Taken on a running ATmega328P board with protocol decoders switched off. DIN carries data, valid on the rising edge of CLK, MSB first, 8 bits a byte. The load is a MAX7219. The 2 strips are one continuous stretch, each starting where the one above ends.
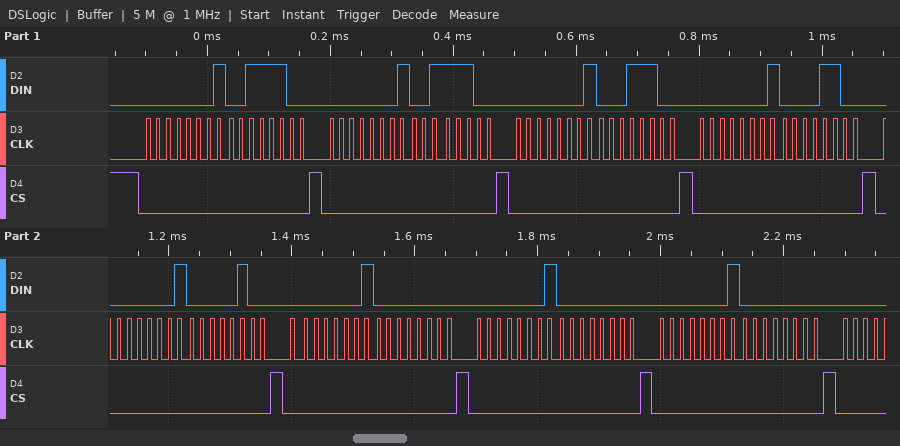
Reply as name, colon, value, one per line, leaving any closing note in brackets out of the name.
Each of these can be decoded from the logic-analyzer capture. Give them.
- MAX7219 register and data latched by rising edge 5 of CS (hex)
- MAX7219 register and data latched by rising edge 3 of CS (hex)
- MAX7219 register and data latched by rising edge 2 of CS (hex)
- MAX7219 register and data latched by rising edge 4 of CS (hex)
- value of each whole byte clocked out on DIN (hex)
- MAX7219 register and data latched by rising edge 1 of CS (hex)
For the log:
MAX7219 register and data latched by rising edge 5 of CS: register 0x1, data 0x04
MAX7219 register and data latched by rising edge 3 of CS: register 0x1, data 0x1C
MAX7219 register and data latched by rising edge 2 of CS: register 0x1, data 0x3C
MAX7219 register and data latched by rising edge 4 of CS: register 0x1, data 0x0C
value of each whole byte clocked out on DIN: 01 3C 01 3C 01 1C 01 0C 01 04 01 00 01 00 01 00
MAX7219 register and data latched by rising edge 1 of CS: register 0x1, data 0x3C
